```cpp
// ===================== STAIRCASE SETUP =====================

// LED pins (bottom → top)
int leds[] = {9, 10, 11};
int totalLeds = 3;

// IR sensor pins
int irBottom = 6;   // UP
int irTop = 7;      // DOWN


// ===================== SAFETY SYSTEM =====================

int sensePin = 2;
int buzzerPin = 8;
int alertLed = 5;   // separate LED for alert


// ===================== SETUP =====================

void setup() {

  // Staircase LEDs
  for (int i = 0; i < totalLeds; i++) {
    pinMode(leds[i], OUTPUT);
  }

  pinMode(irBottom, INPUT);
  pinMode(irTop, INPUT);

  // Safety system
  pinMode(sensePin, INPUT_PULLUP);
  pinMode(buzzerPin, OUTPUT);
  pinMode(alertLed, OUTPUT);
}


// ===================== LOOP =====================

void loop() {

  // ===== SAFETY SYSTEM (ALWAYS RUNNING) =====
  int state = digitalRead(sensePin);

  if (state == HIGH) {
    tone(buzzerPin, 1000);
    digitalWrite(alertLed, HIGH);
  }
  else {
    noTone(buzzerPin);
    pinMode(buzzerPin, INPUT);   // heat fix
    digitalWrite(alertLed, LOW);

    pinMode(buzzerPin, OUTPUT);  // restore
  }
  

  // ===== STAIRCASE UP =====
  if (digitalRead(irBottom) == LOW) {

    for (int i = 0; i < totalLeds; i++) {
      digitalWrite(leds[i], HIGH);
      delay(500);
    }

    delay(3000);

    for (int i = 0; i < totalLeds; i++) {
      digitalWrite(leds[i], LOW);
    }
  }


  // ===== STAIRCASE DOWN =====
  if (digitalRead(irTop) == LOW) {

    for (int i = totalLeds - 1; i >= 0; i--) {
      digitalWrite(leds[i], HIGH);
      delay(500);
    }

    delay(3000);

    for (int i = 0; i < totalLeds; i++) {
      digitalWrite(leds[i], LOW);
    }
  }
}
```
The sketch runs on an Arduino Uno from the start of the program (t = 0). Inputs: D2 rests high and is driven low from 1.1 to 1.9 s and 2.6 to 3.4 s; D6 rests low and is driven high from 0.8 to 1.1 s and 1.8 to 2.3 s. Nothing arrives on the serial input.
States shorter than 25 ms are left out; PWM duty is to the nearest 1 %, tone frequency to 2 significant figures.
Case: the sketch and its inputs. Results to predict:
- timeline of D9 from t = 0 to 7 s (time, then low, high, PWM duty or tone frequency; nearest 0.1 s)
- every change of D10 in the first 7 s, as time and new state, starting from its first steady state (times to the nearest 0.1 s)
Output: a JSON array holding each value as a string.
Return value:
["0 s high; 4.5 s low; 5.5 s high", "0 s low; 0.5 s high; 4.5 s low; 5 s high"]
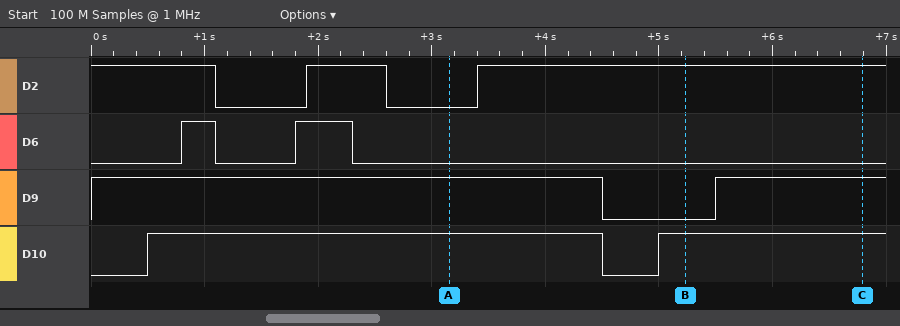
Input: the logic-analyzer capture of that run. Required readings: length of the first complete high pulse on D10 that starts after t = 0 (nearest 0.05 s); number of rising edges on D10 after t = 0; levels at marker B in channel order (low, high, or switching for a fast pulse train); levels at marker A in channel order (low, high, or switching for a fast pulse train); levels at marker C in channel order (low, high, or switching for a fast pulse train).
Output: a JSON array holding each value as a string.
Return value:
["4.00 s", "2", "D2 high, D6 low, D9 low, D10 high", "D2 low, D6 low, D9 high, D10 high", "D2 high, D6 low, D9 high, D10 high"]
